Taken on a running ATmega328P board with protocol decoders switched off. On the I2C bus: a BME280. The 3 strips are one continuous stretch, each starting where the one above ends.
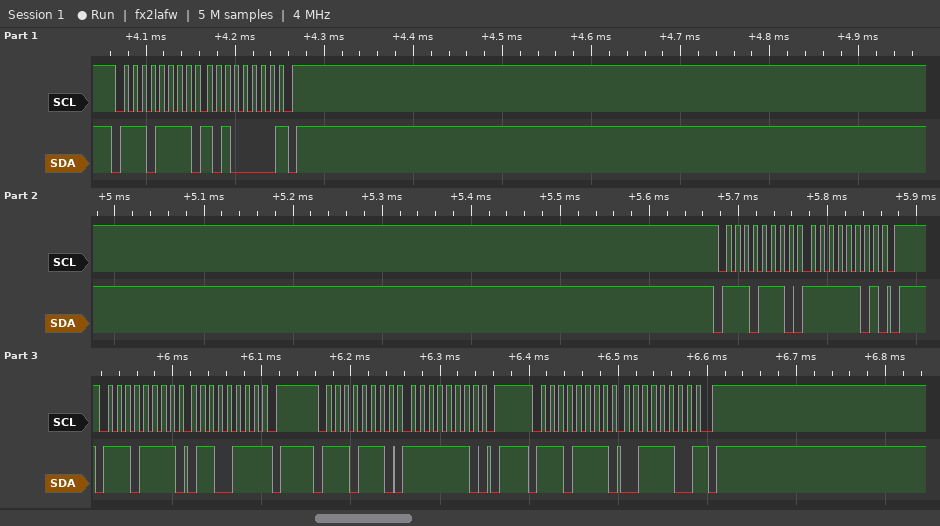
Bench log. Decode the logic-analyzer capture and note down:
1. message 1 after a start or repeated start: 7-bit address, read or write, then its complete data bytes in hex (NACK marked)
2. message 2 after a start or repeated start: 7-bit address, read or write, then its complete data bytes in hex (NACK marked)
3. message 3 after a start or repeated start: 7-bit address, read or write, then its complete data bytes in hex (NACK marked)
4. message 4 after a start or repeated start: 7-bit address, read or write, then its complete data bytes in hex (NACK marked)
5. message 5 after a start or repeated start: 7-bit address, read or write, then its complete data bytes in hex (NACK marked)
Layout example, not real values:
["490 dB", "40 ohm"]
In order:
["0x77 read: A0 NACK", "0x77 write: FD", "0x77 read: 67 NACK", "0x77 write: FE", "0x77 read: 3C NACK"]
